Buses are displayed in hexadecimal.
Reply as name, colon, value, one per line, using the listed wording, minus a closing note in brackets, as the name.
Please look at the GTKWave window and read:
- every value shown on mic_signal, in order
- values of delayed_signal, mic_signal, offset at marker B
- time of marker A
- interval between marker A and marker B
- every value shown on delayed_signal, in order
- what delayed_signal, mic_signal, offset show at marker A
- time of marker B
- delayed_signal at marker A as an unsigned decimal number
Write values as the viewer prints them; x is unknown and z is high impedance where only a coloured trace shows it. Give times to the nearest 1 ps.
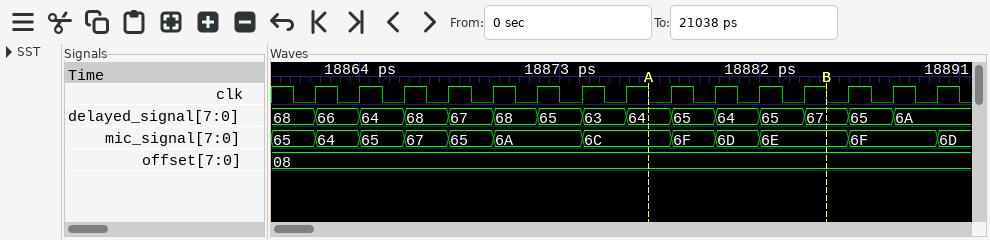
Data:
every value shown on mic_signal, in order: 65, 64, 65, 67, 65, 6A, 6C, 6F, 6D, 6E, 6F, 6D
values of delayed_signal, mic_signal, offset at marker B: delayed_signal=67, mic_signal=6E, offset=08
time of marker A: 18877 ps
interval between marker A and marker B: 8 ps
every value shown on delayed_signal, in order: 68, 66, 64, 68, 67, 68, 65, 63, 64, 65, 64, 65, 67, 65, 6A
what delayed_signal, mic_signal, offset show at marker A: delayed_signal=64, mic_signal=6C, offset=08
time of marker B: 18885 ps
delayed_signal at marker A as an unsigned decimal number: 100
